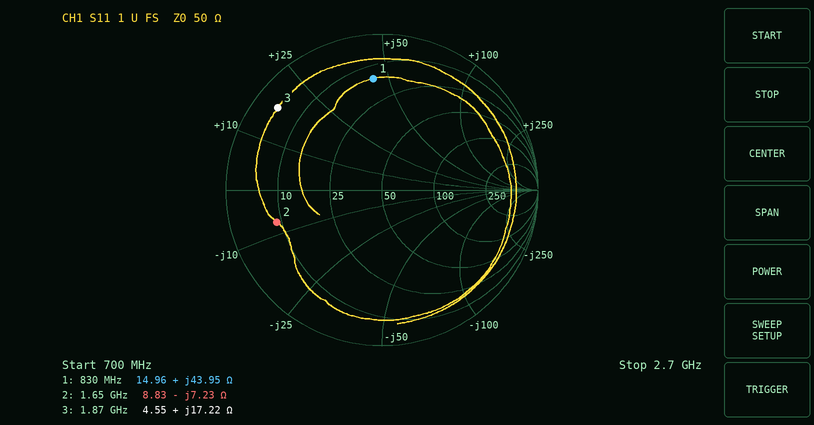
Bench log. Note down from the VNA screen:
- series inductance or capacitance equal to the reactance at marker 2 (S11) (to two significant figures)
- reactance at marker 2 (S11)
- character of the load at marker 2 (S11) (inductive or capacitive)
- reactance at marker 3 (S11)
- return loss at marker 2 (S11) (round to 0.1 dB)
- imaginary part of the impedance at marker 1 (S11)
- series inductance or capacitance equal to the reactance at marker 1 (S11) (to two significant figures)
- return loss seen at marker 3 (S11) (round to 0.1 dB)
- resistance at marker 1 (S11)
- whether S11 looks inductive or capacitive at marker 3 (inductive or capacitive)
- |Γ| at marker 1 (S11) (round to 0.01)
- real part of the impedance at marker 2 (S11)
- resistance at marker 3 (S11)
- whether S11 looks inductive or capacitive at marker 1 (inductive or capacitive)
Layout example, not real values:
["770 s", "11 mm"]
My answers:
["13 pF", "-7.23 Ω", "capacitive", "+17.22 Ω", "3.0 dB", "+43.95 Ω", "8.4 nH", "1.4 dB", "14.96 Ω", "inductive", "0.72", "8.83 Ω", "4.55 Ω", "inductive"]
